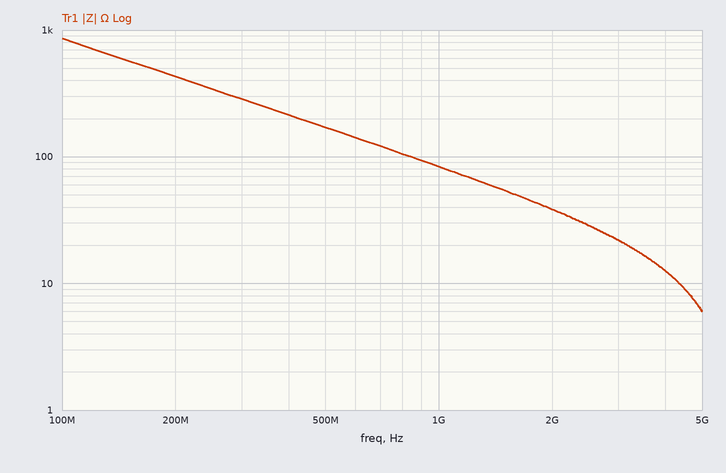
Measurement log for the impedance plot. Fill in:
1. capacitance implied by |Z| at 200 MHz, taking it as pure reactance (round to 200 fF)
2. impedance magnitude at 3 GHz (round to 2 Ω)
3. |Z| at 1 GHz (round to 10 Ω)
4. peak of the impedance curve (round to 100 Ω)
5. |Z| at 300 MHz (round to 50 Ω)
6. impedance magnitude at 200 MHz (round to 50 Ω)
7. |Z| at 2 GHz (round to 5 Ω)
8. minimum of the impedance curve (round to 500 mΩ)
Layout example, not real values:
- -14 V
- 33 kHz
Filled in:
- 1.8 pF
- 22 Ω
- 80 Ω
- 900 Ω
- 300 Ω
- 450 Ω
- 40 Ω
- 6.0 Ω
